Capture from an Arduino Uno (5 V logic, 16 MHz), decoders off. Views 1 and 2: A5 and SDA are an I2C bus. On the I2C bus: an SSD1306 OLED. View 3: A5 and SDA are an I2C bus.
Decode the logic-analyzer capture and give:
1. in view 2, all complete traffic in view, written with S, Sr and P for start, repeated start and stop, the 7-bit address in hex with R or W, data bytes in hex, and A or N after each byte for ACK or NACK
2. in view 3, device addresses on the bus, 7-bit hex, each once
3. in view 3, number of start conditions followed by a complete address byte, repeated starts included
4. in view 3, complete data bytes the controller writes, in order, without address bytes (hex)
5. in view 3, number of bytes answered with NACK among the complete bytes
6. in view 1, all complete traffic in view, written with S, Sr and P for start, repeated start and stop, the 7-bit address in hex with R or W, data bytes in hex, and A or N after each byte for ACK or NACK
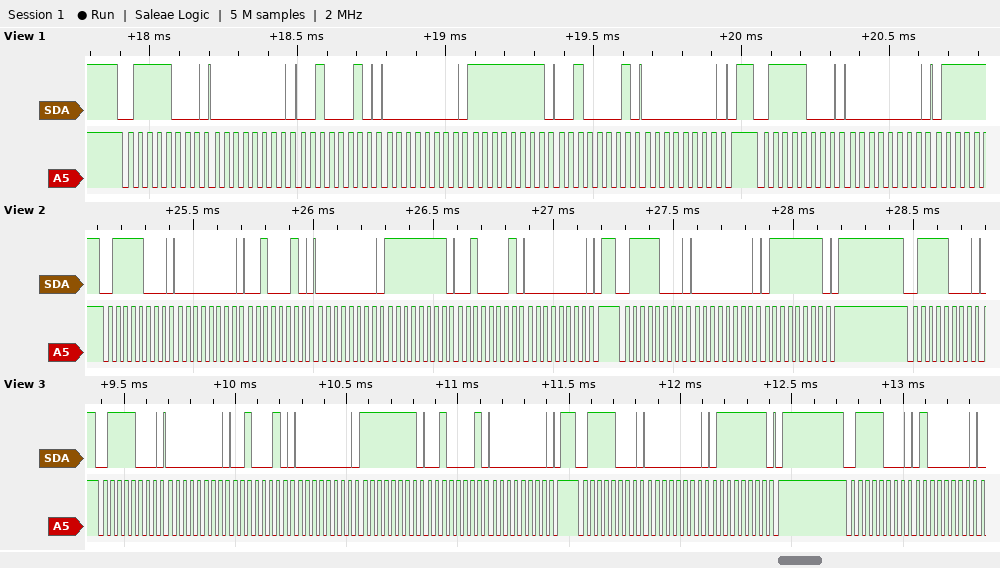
S 3CW A 00 A 22 A 00 A FF A 21 A 00 A P S 3CW A 00 A 7F A P S 3CW A
0x3C
3
00 22 00 FF 21 00 00 7F 40
0
S 3CW A 00 A 22 A 00 A FF A 21 A 00 A P S 3CW A 00 A
